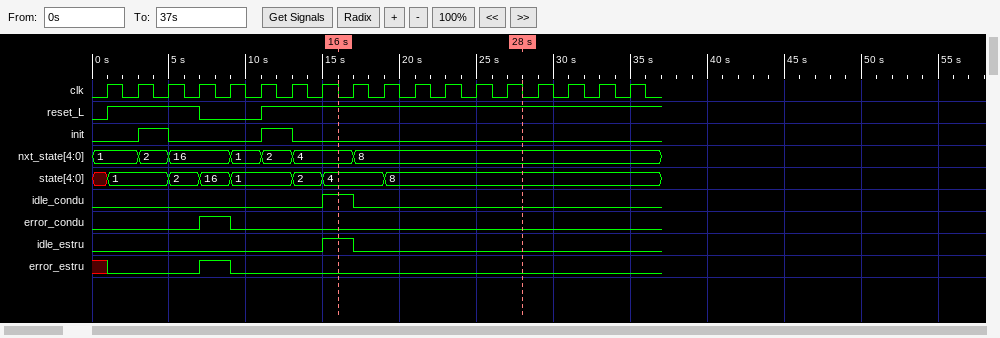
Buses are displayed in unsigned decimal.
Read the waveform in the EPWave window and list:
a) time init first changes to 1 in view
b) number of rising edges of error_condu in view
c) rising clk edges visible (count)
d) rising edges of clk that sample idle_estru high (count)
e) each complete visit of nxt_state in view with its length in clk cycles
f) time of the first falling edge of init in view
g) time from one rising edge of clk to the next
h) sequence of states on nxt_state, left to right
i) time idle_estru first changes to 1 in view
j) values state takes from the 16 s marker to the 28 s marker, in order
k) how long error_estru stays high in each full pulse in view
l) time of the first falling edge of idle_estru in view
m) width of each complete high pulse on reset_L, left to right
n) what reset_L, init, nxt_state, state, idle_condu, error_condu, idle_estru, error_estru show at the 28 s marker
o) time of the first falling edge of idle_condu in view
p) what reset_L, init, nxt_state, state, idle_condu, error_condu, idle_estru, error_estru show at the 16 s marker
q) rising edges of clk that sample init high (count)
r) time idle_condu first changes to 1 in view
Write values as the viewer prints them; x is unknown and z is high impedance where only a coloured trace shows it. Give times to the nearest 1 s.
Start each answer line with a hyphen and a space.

- 3 s
- 1
- 18
- 1
- 2: 1, 16: 2, 1: 1, 2: 1, 4: 2
- 5 s
- 2 s
- 1, 2, 16, 1, 2, 4, 8
- 15 s
- 4, 8
- 2 s
- 17 s
- 6 s
- reset_L=1, init=0, nxt_state=8, state=8, idle_condu=0, error_condu=0, idle_estru=0, error_estru=0
- 17 s
- reset_L=1, init=0, nxt_state=4, state=4, idle_condu=1, error_condu=0, idle_estru=1, error_estru=0
- 2
- 15 s
